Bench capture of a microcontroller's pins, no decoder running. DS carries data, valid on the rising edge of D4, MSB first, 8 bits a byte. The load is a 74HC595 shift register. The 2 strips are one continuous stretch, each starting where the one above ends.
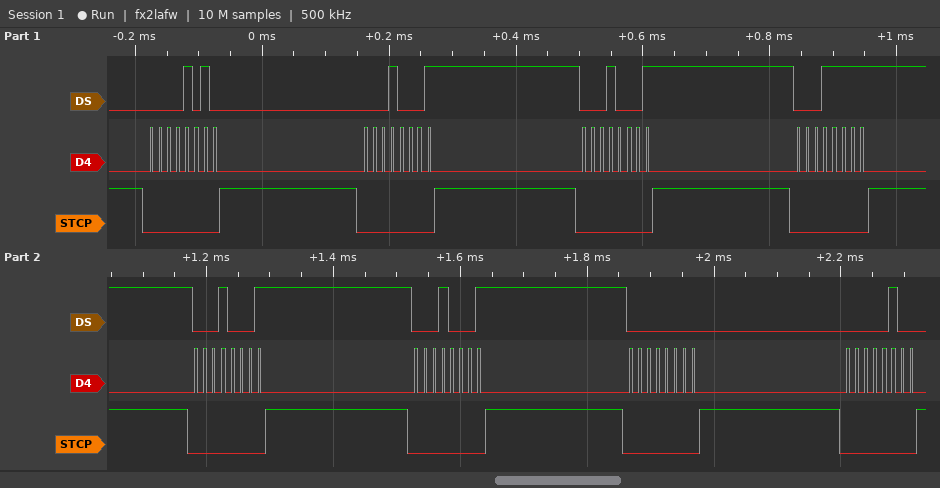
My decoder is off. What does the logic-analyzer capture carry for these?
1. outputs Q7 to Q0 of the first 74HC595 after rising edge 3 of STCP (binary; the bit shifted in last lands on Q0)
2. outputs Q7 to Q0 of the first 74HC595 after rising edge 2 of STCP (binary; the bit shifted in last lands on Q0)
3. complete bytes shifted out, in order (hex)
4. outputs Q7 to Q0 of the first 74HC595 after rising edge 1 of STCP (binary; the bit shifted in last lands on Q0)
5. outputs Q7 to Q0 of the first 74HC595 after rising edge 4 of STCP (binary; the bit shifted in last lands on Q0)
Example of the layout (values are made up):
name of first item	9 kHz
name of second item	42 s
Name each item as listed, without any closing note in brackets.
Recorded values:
outputs Q7 to Q0 of the first 74HC595 after rising edge 3 of STCP	00010001
outputs Q7 to Q0 of the first 74HC595 after rising edge 2 of STCP	00010001
complete bytes shifted out, in order	0A 11 11 1F 11 11 00 04
outputs Q7 to Q0 of the first 74HC595 after rising edge 1 of STCP	00001010
outputs Q7 to Q0 of the first 74HC595 after rising edge 4 of STCP	00011111
